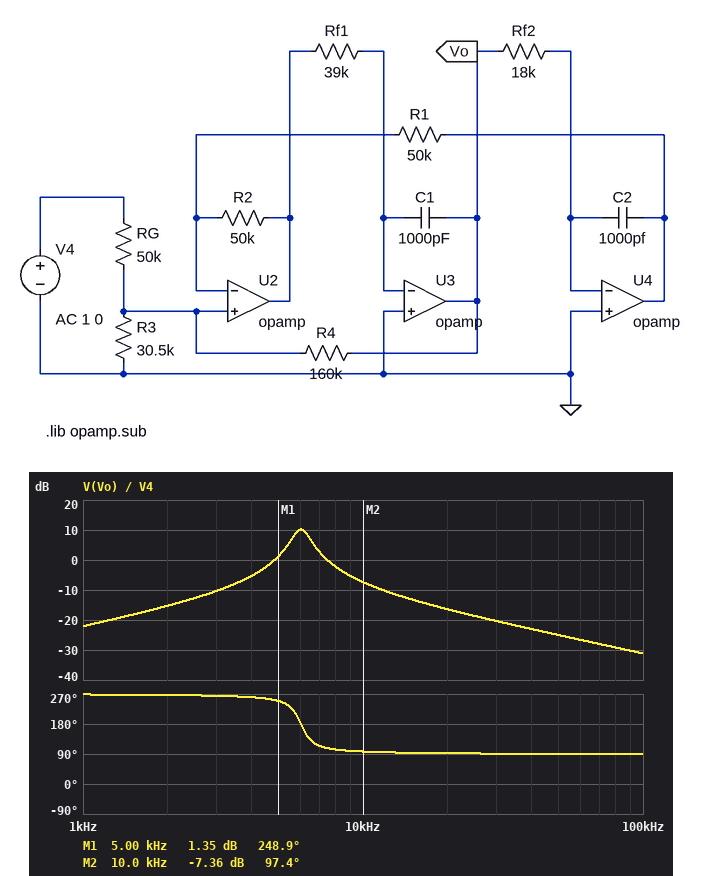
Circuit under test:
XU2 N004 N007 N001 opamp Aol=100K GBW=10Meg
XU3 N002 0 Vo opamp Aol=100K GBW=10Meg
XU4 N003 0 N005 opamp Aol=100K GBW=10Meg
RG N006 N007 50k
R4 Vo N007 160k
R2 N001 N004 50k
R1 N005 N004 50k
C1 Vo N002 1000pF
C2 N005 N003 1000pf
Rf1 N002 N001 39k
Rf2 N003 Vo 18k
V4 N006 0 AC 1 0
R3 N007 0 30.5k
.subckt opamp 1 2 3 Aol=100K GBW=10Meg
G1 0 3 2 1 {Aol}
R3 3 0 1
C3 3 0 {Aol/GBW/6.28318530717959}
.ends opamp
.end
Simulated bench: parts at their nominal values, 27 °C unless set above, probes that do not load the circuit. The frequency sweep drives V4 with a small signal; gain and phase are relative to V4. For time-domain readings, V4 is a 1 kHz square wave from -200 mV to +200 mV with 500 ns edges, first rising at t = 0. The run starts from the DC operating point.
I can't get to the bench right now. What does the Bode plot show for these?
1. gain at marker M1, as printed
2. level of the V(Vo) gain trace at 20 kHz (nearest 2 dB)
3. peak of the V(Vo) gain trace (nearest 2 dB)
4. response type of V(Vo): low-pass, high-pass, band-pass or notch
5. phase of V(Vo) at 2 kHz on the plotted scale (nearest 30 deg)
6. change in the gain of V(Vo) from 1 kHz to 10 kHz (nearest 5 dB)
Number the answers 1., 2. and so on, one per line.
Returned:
1. 1.35 dB
2. -16 dB
3. 10 dB
4. band-pass
5. 270 deg
6. 15 dB
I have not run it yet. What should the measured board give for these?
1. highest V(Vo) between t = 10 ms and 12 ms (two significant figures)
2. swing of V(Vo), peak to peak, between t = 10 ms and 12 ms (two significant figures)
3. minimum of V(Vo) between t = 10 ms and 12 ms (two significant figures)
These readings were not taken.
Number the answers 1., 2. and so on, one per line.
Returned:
1. 130 mV
2. 260 mV
3. -130 mV
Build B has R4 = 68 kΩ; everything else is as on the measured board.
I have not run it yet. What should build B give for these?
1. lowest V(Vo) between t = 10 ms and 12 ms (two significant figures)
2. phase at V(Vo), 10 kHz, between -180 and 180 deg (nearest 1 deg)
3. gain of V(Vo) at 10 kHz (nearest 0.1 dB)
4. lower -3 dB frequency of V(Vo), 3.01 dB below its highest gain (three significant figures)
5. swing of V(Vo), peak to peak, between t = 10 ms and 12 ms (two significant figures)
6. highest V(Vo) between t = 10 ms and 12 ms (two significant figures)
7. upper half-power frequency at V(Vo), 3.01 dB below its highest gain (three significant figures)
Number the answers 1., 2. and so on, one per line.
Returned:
1. -120 mV
2. 105 deg
3. -8.8 dB
4. 5.19 kHz
5. 250 mV
6. 120 mV
7. 6.95 kHz
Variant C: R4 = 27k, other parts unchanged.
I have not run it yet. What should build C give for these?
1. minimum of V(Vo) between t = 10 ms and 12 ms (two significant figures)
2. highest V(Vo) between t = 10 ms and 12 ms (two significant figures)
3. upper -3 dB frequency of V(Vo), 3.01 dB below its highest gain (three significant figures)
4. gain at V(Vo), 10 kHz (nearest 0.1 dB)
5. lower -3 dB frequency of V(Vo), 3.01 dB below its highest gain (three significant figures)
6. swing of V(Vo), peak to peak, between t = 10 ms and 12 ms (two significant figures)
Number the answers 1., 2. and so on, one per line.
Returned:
1. -83 mV
2. 83 mV
3. 7.91 kHz
4. -12.0 dB
5. 4.56 kHz
6. 170 mV
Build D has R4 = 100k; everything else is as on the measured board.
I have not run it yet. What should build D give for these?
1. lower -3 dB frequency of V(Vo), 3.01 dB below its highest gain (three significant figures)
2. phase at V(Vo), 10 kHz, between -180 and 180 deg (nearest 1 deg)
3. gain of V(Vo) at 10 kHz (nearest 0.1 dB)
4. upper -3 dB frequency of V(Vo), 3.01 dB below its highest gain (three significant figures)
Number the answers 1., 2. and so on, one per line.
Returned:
1. 5.40 kHz
2. 101 deg
3. -8.0 dB
4. 6.68 kHz
